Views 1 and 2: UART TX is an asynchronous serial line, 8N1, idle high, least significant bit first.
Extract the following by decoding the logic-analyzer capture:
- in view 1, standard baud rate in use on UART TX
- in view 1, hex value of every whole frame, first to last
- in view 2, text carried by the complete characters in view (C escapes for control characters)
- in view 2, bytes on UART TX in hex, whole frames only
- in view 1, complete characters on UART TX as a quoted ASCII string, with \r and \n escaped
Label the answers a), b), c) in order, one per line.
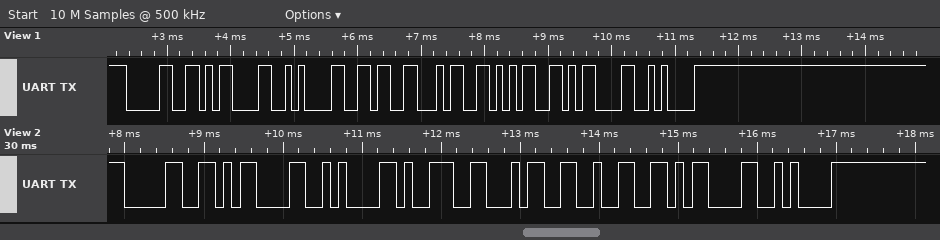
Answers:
a) 9600 baud
b) 0x30 0x0D 0x0A 0x36 0x34 0x35 0x0D 0x0A
c) "0\r\n942\r\n"
d) 30 0D 0A 39 34 32 0D 0A
e) "0\r\n645\r\n"
